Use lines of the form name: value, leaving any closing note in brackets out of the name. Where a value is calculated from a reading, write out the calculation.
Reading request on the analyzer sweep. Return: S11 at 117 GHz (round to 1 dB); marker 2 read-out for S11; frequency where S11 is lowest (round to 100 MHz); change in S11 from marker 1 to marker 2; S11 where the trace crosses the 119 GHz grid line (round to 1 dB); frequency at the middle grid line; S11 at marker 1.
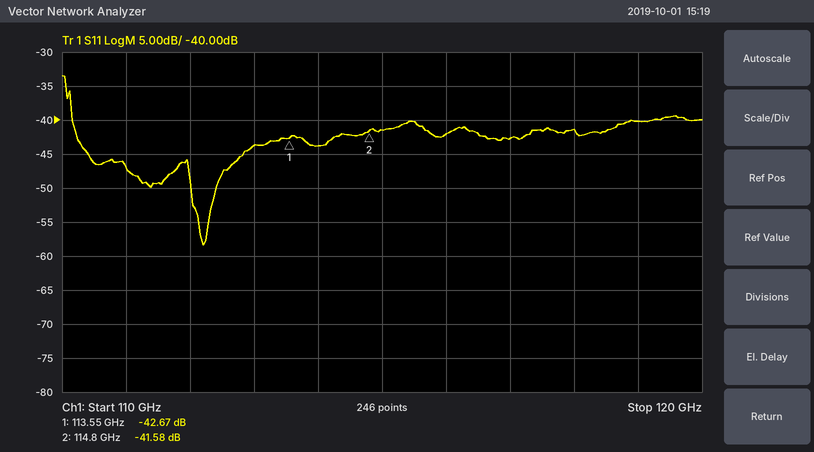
S11 at 117 GHz: -43 dB
marker 2 read-out for S11: -41.58 dB
frequency where S11 is lowest: 112.2 GHz
change in S11 from marker 1 to marker 2: -41.58 − (-42.67) = 1.09 dB
S11 where the trace crosses the 119 GHz grid line: -40 dB
frequency at the middle grid line: 115 GHz
S11 at marker 1: -42.67 dB
